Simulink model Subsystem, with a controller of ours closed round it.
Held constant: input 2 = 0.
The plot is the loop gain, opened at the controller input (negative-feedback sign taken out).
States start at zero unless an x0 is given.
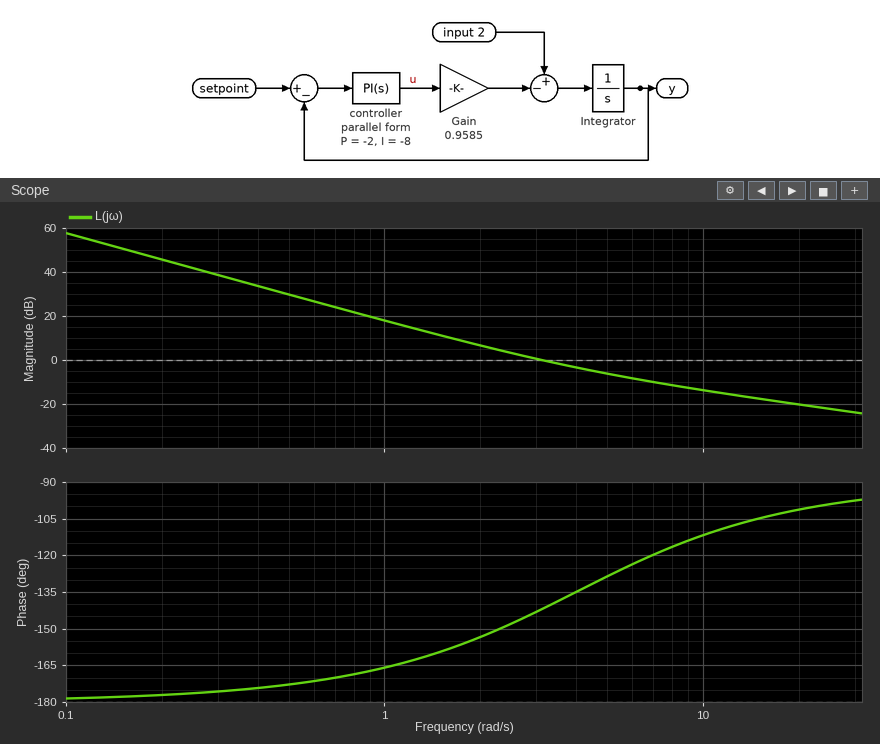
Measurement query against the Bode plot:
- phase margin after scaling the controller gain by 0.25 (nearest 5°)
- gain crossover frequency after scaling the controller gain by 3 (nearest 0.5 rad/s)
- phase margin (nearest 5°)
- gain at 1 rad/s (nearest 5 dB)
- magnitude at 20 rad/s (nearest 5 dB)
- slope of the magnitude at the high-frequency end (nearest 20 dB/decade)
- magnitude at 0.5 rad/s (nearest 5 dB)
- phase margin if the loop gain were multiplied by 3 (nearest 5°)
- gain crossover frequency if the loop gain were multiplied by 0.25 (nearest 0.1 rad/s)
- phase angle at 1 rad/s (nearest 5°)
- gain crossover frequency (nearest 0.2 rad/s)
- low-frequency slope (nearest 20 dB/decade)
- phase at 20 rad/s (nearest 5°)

20°
6.5 rad/s
40°
20 dB
-20 dB
-20 dB/decade
30 dB
60°
1.4 rad/s
-165°
3.2 rad/s
-40 dB/decade
-100°
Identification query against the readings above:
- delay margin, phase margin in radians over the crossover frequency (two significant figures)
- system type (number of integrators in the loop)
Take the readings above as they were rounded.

0.22 s
2
